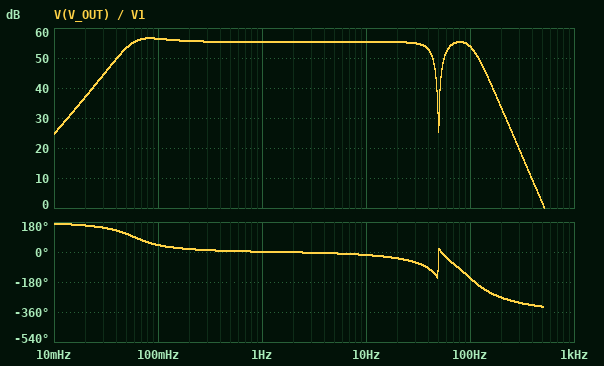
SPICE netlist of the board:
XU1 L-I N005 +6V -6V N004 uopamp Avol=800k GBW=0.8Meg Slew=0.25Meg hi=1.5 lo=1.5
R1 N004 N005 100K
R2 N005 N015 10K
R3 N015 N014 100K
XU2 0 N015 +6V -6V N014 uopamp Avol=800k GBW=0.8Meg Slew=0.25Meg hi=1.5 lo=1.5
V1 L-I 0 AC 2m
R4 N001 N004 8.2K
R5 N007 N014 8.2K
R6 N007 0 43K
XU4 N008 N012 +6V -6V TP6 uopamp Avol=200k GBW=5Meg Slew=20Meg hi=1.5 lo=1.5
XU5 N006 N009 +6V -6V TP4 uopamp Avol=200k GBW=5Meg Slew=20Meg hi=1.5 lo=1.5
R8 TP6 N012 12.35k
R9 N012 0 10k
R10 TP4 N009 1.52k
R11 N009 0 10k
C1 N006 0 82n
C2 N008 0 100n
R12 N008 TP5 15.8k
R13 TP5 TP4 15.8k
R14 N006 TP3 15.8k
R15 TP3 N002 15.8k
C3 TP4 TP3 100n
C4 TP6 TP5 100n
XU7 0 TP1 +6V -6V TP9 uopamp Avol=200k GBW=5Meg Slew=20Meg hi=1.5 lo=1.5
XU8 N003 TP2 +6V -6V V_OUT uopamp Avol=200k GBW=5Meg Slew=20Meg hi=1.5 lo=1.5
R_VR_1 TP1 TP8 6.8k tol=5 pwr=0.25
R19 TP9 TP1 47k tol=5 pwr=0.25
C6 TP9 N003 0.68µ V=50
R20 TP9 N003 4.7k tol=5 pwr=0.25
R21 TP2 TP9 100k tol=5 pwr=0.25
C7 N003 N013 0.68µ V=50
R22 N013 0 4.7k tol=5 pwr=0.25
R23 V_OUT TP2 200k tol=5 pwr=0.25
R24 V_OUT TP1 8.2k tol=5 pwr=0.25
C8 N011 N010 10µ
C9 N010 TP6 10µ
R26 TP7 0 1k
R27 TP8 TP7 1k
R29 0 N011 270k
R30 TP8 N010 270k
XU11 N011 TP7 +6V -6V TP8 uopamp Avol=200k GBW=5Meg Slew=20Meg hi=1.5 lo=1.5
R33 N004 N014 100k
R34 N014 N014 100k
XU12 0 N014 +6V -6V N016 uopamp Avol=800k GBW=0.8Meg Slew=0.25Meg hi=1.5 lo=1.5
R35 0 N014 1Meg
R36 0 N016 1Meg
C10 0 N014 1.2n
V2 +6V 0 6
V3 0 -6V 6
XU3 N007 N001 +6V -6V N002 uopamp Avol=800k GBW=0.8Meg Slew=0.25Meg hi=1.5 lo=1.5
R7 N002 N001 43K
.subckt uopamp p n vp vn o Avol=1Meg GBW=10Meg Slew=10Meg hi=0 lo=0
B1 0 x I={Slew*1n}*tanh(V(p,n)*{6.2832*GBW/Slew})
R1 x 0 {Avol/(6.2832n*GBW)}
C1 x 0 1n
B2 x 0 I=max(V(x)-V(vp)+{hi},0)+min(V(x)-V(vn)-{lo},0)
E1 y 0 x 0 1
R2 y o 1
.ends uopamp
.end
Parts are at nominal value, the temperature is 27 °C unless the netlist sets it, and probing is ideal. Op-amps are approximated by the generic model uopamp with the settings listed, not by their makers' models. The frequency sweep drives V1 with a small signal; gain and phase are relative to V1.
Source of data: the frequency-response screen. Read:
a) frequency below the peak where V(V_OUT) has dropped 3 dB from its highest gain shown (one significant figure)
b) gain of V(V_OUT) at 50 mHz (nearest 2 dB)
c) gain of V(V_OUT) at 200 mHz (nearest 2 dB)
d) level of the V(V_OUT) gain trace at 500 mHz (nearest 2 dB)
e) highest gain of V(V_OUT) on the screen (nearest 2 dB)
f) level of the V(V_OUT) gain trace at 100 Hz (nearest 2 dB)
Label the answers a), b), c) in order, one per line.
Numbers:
a) 50 mHz
b) 54 dB
c) 56 dB
d) 56 dB
e) 56 dB
f) 54 dB
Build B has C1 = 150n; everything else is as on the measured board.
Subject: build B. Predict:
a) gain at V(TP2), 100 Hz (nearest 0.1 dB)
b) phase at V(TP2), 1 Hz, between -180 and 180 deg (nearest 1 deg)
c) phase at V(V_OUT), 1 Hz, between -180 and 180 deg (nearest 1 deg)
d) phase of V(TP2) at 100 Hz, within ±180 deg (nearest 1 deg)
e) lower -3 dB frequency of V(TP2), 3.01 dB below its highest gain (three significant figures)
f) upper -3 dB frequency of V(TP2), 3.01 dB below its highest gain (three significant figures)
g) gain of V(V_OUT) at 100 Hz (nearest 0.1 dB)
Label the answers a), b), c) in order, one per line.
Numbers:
a) 52.6 dB
b) 3 deg
c) 1 deg
d) 135 deg
e) 38.0 Hz
f) 60.7 Hz
g) 48.2 dB
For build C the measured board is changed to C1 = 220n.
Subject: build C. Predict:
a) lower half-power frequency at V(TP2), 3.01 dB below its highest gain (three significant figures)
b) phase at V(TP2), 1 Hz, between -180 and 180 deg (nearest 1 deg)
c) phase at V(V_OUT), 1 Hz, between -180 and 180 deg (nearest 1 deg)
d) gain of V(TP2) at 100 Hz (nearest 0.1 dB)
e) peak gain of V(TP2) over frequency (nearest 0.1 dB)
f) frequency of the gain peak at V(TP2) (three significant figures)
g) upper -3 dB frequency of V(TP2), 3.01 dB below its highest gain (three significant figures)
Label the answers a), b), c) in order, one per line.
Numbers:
a) 36.6 Hz
b) 2 deg
c) 0 deg
d) 48.9 dB
e) 63.2 dB
f) 48.4 Hz
g) 59.8 Hz
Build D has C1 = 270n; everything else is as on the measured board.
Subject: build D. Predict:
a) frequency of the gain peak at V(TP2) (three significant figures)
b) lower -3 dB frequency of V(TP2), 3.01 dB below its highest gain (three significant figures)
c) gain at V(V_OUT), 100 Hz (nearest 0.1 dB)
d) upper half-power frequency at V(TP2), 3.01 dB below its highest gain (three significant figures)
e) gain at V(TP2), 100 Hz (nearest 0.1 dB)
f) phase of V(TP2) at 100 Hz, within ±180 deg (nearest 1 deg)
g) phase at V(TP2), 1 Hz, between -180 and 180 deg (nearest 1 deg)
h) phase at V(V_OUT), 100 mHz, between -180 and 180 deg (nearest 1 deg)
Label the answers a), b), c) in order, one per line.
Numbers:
a) 48.2 Hz
b) 35.9 Hz
c) 42.6 dB
d) 59.5 Hz
e) 47.0 dB
f) 127 deg
g) 2 deg
h) 42 deg
